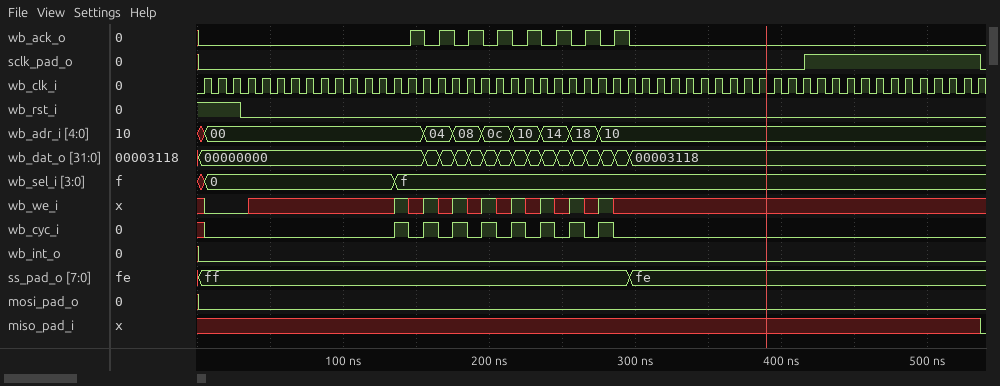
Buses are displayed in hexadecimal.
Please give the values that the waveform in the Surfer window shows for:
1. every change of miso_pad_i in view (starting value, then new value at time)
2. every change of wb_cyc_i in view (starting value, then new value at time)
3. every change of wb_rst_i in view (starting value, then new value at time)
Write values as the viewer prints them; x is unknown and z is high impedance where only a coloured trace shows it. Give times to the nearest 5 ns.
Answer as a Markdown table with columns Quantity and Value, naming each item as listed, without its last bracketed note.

| Quantity | Value |
|---|---|
| every change of miso_pad_i in view | x, 0 at 535 ns |
| every change of wb_cyc_i in view | x, 0 at 5 ns, 1 at 135 ns, 0 at 145 ns, 1 at 155 ns, 0 at 165 ns, 1 at 175 ns, 0 at 185 ns, 1 at 195 ns, 0 at 205 ns, 1 at 215 ns, 0 at 225 ns, 1 at 235 ns, 0 at 245 ns, 1 at 255 ns, 0 at 265 ns, 1 at 275 ns, 0 at 285 ns |
| every change of wb_rst_i in view | 1, 0 at 30 ns |
